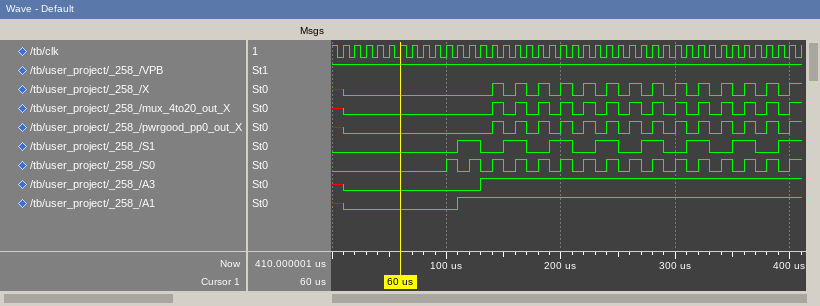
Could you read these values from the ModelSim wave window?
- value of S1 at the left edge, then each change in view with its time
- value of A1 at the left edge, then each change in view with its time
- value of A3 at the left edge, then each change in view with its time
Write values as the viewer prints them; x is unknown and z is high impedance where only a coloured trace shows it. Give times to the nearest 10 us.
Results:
0, 1 at 110 us, 0 at 130 us, 1 at 150 us, 0 at 170 us, 1 at 190 us, 0 at 210 us, 1 at 230 us, 0 at 250 us, 1 at 270 us, 0 at 290 us, 1 at 310 us, 0 at 330 us, 1 at 350 us, 0 at 370 us, 1 at 390 us
x, 0 at 10 us, 1 at 110 us
x, 0 at 10 us, 1 at 130 us
